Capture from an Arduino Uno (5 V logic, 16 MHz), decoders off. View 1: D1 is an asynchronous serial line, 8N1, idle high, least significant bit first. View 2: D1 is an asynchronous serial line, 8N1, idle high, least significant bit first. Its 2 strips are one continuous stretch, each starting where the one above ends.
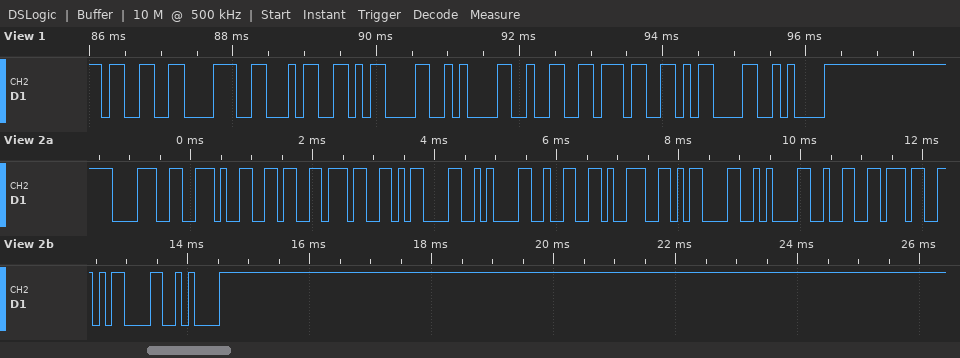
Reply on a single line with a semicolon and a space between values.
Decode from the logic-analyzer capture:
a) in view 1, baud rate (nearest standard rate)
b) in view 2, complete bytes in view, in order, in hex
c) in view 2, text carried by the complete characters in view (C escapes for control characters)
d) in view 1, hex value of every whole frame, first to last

9600 baud; 38 2E 36 37 0D 0A 32 39 0D 0A 32 37 0D 0A; "8.67\r\n29\r\n27\r\n"; 33 38 34 0D 0A 32 37 0D 0A
